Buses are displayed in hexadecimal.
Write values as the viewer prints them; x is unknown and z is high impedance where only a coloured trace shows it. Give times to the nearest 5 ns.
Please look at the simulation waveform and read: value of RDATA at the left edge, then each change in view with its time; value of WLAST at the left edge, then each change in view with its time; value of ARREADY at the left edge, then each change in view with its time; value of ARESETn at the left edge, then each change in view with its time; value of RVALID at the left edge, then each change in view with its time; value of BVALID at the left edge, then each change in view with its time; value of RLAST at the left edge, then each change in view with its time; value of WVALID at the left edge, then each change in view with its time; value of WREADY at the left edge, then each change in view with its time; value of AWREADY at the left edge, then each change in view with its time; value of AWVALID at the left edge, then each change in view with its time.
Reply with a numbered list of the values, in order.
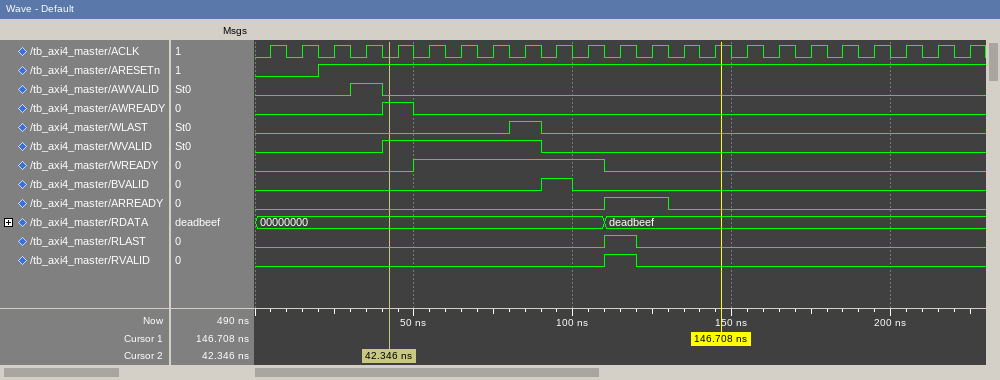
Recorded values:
1. 00000000, deadbeef at 110 ns
2. 0, 1 at 80 ns, 0 at 90 ns
3. 0, 1 at 110 ns, 0 at 130 ns
4. 0, 1 at 20 ns
5. 0, 1 at 110 ns, 0 at 120 ns
6. 0, 1 at 90 ns, 0 at 100 ns
7. 0, 1 at 110 ns, 0 at 120 ns
8. 0, 1 at 40 ns, 0 at 90 ns
9. 0, 1 at 50 ns, 0 at 110 ns
10. 0, 1 at 40 ns, 0 at 50 ns
11. 0, 1 at 30 ns, 0 at 40 ns
